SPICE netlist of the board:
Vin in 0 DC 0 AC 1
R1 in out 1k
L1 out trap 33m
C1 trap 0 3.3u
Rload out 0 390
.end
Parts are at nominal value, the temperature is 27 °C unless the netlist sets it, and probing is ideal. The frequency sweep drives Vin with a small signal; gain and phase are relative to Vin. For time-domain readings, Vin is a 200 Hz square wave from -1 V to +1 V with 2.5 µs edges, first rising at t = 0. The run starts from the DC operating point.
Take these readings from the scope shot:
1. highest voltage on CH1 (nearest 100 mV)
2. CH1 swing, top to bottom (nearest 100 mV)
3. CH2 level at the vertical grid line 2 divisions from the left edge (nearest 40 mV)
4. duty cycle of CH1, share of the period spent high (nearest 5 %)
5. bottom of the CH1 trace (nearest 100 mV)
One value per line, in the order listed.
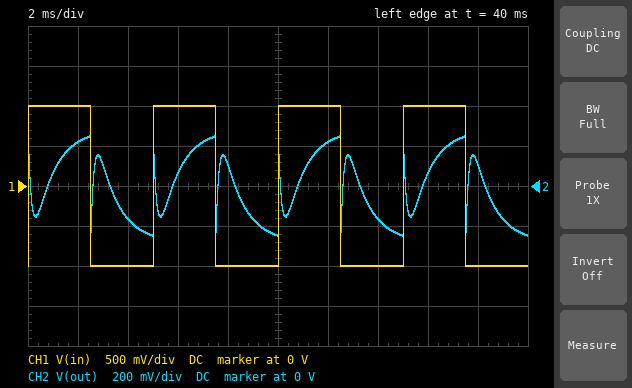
1.0 V
2.0 V
-160 mV
50 %
-1.0 V
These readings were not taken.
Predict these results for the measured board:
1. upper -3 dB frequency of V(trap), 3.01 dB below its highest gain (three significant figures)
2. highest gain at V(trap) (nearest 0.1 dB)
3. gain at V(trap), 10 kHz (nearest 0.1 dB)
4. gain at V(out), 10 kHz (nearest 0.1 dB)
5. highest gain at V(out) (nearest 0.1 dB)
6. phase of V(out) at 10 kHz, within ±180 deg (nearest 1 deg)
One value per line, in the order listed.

196 Hz
-11.0 dB
-63.8 dB
-11.1 dB
-11.0 dB
8 deg
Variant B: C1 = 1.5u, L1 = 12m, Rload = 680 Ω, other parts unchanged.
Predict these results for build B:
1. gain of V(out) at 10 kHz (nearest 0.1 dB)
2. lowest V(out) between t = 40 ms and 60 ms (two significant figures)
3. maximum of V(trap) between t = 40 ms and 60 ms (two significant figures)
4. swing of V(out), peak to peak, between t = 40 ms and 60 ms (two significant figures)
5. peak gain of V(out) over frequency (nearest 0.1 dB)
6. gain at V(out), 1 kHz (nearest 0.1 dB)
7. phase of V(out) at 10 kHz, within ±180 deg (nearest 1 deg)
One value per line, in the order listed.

-9.0 dB
-390 mV
390 mV
790 mV
-7.9 dB
-30.3 dB
29 deg
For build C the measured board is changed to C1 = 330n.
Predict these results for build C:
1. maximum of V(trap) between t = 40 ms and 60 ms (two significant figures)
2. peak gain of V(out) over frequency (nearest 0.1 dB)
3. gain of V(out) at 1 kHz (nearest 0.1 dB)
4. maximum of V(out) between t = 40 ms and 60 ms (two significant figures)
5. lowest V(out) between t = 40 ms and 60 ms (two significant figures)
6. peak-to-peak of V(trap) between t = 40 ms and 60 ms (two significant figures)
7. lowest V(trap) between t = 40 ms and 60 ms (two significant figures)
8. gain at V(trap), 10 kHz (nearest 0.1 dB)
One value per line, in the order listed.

400 mV
-11.0 dB
-14.1 dB
340 mV
-340 mV
800 mV
-400 mV
-43.6 dB
